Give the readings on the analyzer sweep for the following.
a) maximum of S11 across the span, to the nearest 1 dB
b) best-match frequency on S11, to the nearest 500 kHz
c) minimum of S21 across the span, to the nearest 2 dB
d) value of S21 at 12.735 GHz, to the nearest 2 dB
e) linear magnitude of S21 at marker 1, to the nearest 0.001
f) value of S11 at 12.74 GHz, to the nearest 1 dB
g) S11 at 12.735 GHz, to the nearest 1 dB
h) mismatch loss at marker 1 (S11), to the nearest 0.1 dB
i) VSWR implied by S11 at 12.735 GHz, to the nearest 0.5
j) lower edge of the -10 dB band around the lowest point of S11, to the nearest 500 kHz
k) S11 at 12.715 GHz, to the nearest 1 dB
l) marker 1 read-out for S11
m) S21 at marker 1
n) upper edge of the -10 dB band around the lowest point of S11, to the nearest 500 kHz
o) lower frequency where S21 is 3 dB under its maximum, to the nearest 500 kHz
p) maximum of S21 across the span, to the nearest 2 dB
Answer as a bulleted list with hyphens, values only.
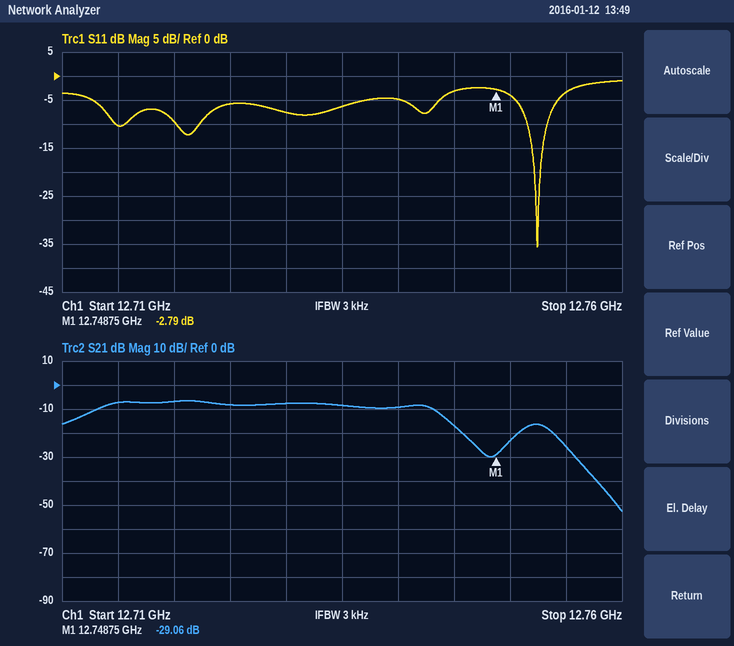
- -1 dB
- 12.7525 GHz
- -52 dB
- -8 dB
- 0.035
- -5 dB
- -6 dB
- 3.2 dB
- 3.0
- 12.7515 GHz
- -10 dB
- -2.79 dB
- -29.06 dB
- 12.7535 GHz
- 12.7135 GHz
- -6 dB
